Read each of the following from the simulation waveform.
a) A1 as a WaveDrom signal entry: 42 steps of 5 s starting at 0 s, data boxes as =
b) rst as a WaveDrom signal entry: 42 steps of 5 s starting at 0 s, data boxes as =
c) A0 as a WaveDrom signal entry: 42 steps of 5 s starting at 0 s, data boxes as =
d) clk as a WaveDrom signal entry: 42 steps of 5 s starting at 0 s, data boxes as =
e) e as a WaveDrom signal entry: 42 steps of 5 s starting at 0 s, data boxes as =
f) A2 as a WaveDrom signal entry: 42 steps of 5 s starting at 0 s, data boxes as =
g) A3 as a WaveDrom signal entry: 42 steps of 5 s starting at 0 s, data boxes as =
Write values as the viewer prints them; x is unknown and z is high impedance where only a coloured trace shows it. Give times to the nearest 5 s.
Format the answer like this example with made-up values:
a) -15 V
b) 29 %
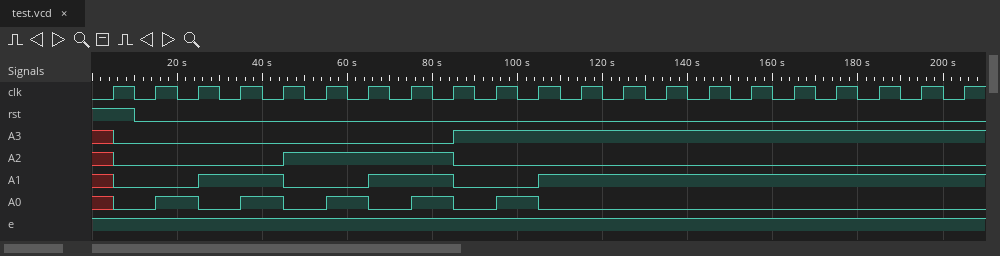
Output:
a) {name: 'A1', wave: 'x0...1...0...1...0...1....................'}
b) {name: 'rst', wave: '1.0.......................................'}
c) {name: 'A0', wave: 'x0.1.0.1.0.1.0.1.0.1.0....................'}
d) {name: 'clk', wave: '010101010101010101010101010101010101010101'}
e) {name: 'e', wave: '1.........................................'}
f) {name: 'A2', wave: 'x0.......1.......0........................'}
g) {name: 'A3', wave: 'x0...............1........................'}
